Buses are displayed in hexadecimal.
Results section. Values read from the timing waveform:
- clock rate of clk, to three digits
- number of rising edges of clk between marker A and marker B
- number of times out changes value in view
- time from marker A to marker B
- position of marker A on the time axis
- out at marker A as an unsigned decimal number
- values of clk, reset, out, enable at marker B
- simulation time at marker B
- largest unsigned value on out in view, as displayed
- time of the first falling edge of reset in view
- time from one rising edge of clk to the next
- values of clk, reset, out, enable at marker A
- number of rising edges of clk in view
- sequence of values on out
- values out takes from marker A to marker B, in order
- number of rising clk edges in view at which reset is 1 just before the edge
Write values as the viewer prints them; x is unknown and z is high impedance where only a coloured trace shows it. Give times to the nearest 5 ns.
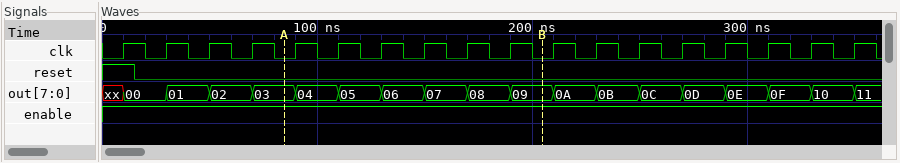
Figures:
50.0 MHz
6
18
120 ns
85 ns
3
clk=0, reset=0, out=09, enable=1
205 ns
11
15 ns
20 ns
clk=0, reset=0, out=03, enable=1
18
xx, 00, 01, 02, 03, 04, 05, 06, 07, 08, 09, 0A, 0B, 0C, 0D, 0E, 0F, 10, 11
03, 04, 05, 06, 07, 08, 09
1
